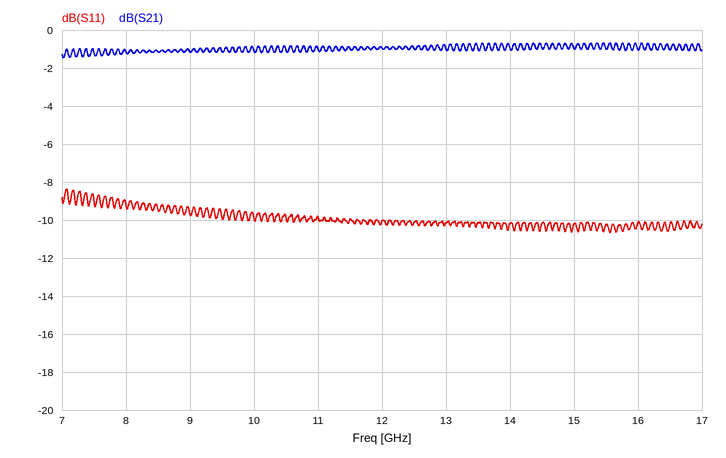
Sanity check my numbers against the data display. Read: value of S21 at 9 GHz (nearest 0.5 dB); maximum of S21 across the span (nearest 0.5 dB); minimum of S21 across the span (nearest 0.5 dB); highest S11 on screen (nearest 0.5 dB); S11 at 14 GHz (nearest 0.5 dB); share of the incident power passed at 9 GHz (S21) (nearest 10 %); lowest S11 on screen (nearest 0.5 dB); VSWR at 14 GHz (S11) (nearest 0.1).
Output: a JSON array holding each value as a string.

["-1.0 dB", "-0.5 dB", "-1.5 dB", "-8.5 dB", "-10.0 dB", "80 %", "-10.5 dB", "1.9"]
